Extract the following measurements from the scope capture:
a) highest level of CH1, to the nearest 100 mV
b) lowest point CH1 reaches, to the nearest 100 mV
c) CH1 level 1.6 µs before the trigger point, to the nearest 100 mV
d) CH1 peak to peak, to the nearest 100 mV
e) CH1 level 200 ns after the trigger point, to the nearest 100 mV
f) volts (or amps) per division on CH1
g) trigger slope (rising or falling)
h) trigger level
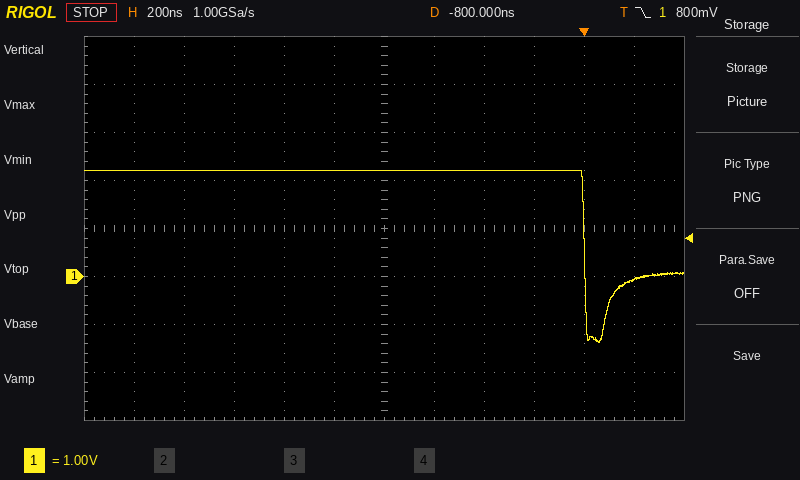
2.2 V
-1.4 V
2.2 V
3.6 V
-100 mV
1 V
falling
800 mV
